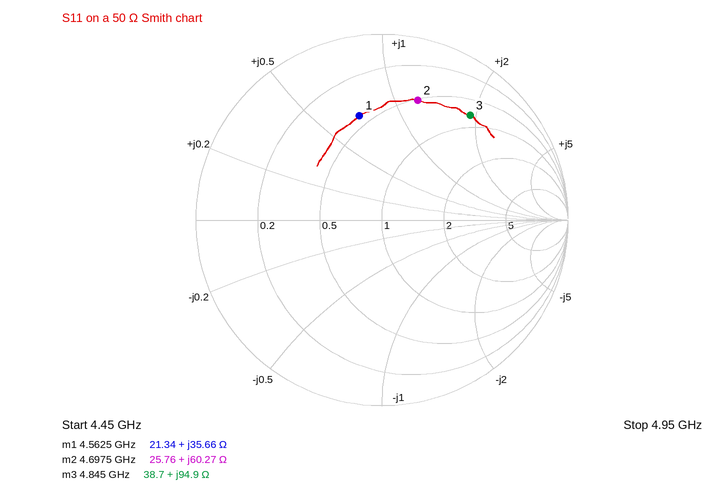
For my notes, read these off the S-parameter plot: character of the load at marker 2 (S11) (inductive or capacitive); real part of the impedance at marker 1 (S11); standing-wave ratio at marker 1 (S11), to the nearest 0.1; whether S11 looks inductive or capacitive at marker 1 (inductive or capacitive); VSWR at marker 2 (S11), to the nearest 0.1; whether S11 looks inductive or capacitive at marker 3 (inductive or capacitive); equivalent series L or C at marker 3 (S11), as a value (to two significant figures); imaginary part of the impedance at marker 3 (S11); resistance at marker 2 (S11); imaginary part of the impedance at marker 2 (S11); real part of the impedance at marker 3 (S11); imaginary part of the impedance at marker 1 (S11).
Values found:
inductive
21.34 Ω
3.7
inductive
5.1
inductive
3.1 nH
+94.9 Ω
25.76 Ω
+60.27 Ω
38.7 Ω
+35.66 Ω
